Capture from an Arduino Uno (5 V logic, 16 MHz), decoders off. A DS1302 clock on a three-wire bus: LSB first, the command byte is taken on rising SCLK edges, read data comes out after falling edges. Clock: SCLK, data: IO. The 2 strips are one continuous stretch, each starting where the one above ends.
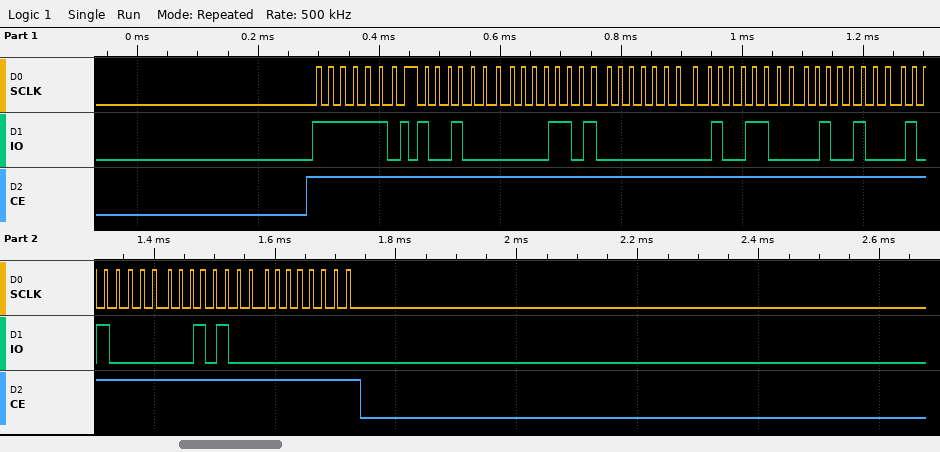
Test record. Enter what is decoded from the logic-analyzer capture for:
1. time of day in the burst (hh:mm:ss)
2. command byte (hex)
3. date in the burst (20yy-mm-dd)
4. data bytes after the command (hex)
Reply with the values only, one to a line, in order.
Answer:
00:58:09
0xBF
2014-12-19
09 58 00 19 12 05 14 00
